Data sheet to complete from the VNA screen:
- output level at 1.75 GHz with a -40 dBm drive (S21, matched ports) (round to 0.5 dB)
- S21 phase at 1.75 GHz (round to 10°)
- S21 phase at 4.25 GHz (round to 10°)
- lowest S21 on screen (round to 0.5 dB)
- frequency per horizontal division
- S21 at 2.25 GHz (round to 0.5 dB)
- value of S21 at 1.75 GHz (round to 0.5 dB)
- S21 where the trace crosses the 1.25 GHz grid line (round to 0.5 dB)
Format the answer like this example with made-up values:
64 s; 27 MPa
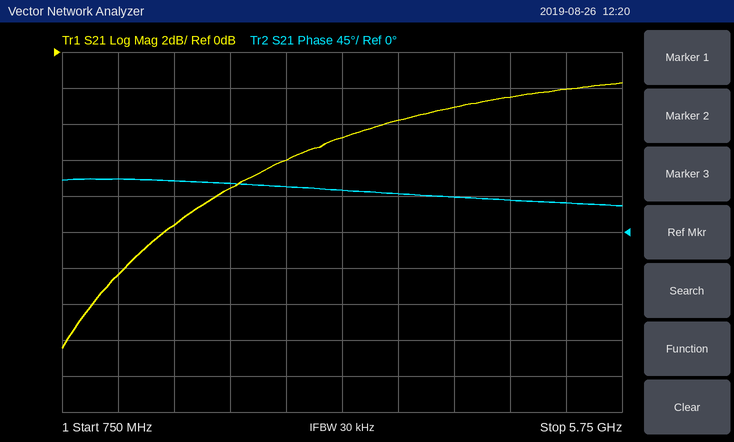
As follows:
-49.5 dBm; 60°; 40°; -16.5 dB; 500 MHz; -7.5 dB; -9.5 dB; -12.5 dB
